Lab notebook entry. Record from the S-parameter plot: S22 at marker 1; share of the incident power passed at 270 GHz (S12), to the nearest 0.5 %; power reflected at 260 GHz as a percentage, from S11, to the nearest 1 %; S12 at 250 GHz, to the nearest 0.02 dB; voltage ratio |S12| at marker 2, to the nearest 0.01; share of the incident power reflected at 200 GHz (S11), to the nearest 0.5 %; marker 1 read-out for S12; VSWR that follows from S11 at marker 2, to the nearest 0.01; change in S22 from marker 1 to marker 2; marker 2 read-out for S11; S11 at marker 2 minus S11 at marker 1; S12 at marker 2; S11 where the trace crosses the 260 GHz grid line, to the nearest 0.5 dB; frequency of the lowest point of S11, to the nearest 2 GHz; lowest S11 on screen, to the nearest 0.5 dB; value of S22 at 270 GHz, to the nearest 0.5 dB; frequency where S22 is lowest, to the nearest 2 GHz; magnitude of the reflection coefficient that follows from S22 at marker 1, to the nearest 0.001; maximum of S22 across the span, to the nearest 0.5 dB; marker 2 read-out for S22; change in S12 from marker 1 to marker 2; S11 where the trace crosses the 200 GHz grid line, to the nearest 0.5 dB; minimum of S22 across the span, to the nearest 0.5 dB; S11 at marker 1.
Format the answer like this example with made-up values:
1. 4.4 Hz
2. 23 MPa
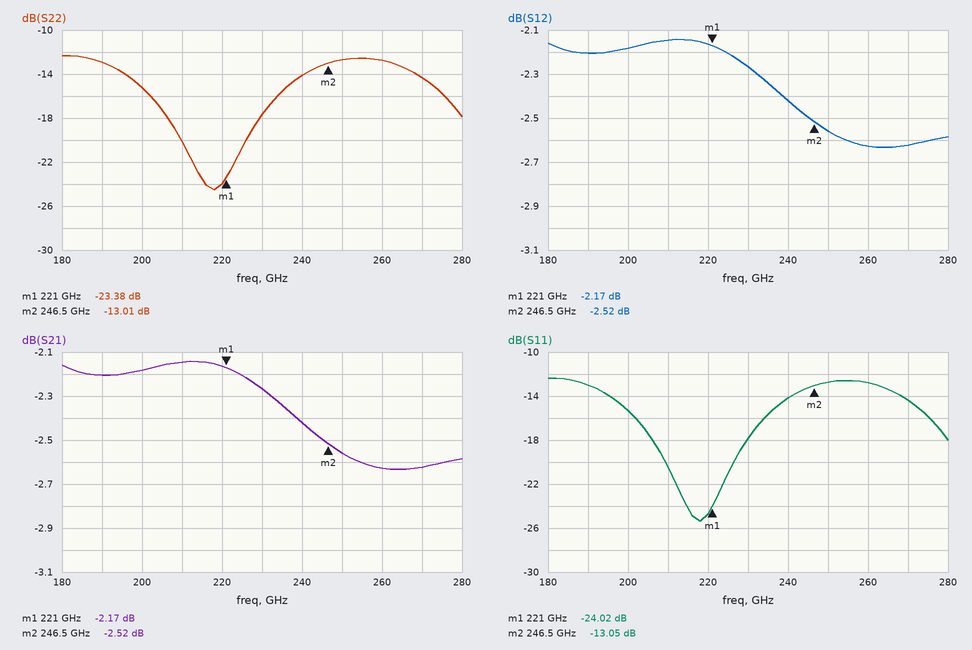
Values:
1. -23.38 dB
2. 54.5 %
3. 5 %
4. -2.56 dB
5. 0.75
6. 3.0 %
7. -2.17 dB
8. 1.57
9. 10.37 dB
10. -13.05 dB
11. 10.97 dB
12. -2.52 dB
13. -13.0 dB
14. 218 GHz
15. -25.5 dB
16. -14.5 dB
17. 218 GHz
18. 0.068
19. -12.5 dB
20. -13.01 dB
21. -0.35 dB
22. -15.5 dB
23. -24.5 dB
24. -24.02 dB
